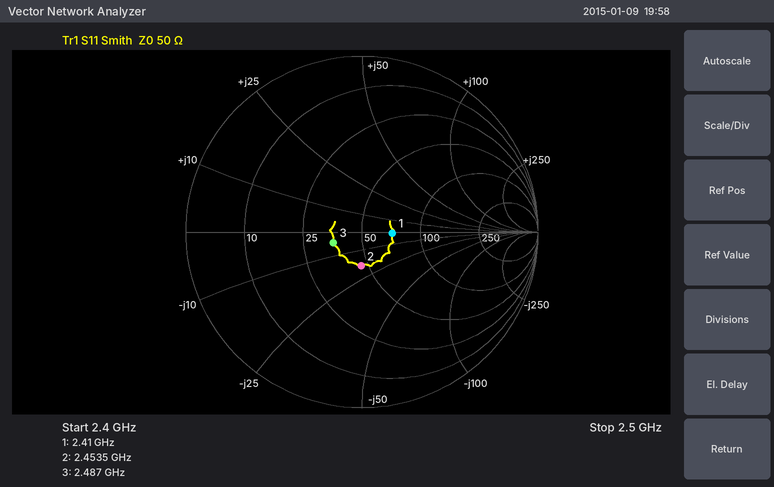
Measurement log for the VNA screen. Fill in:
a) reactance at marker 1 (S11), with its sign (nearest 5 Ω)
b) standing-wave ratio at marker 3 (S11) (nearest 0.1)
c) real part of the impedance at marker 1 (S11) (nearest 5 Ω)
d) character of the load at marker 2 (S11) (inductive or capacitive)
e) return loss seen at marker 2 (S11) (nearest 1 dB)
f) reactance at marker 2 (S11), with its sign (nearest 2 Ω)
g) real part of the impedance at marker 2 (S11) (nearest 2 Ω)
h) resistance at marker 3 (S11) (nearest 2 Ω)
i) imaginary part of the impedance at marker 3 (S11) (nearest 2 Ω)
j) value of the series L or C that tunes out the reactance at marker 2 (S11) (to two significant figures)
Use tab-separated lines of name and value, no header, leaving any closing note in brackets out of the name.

reactance at marker 1 (S11), with its sign	0 Ω
standing-wave ratio at marker 3 (S11)	1.4
real part of the impedance at marker 1 (S11)	70 Ω
character of the load at marker 2 (S11)	capacitive
return loss seen at marker 2 (S11)	14 dB
reactance at marker 2 (S11), with its sign	-18 Ω
real part of the impedance at marker 2 (S11)	46 Ω
resistance at marker 3 (S11)	36 Ω
imaginary part of the impedance at marker 3 (S11)	-4 Ω
value of the series L or C that tunes out the reactance at marker 2 (S11)	1.2 nH
